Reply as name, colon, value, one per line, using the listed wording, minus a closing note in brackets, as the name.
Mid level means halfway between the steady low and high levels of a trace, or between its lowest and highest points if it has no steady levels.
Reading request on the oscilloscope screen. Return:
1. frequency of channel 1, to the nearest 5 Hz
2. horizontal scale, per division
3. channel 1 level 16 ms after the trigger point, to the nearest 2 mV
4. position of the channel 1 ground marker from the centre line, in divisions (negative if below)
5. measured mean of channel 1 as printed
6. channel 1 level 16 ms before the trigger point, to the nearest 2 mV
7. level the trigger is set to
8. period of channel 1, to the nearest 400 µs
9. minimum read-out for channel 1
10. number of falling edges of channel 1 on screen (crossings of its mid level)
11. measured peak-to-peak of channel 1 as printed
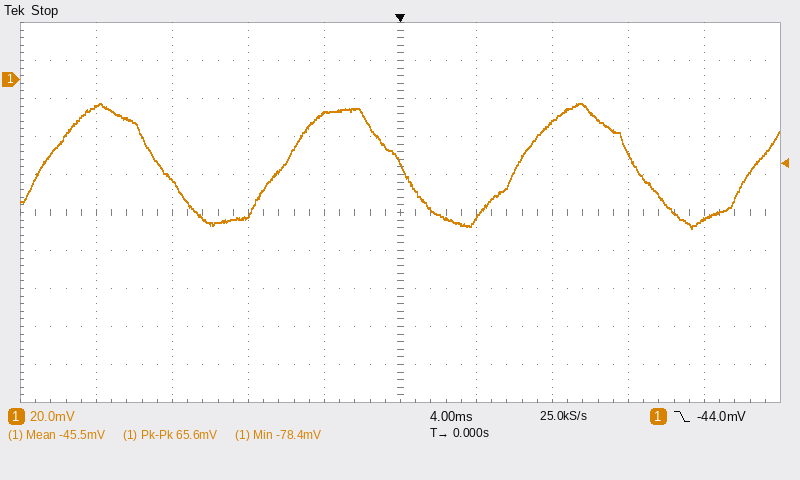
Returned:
frequency of channel 1, to the nearest 5 Hz: 80 Hz
horizontal scale, per division: 4 ms
channel 1 level 16 ms after the trigger point, to the nearest 2 mV: -74 mV
position of the channel 1 ground marker from the centre line, in divisions: +3.5 div
measured mean of channel 1 as printed: -45.5 mV
channel 1 level 16 ms before the trigger point, to the nearest 2 mV: -14 mV
level the trigger is set to: -44.0 mV
period of channel 1, to the nearest 400 µs: 12.4 ms
minimum read-out for channel 1: -78.4 mV
number of falling edges of channel 1 on screen: 3
measured peak-to-peak of channel 1 as printed: 65.6 mV
